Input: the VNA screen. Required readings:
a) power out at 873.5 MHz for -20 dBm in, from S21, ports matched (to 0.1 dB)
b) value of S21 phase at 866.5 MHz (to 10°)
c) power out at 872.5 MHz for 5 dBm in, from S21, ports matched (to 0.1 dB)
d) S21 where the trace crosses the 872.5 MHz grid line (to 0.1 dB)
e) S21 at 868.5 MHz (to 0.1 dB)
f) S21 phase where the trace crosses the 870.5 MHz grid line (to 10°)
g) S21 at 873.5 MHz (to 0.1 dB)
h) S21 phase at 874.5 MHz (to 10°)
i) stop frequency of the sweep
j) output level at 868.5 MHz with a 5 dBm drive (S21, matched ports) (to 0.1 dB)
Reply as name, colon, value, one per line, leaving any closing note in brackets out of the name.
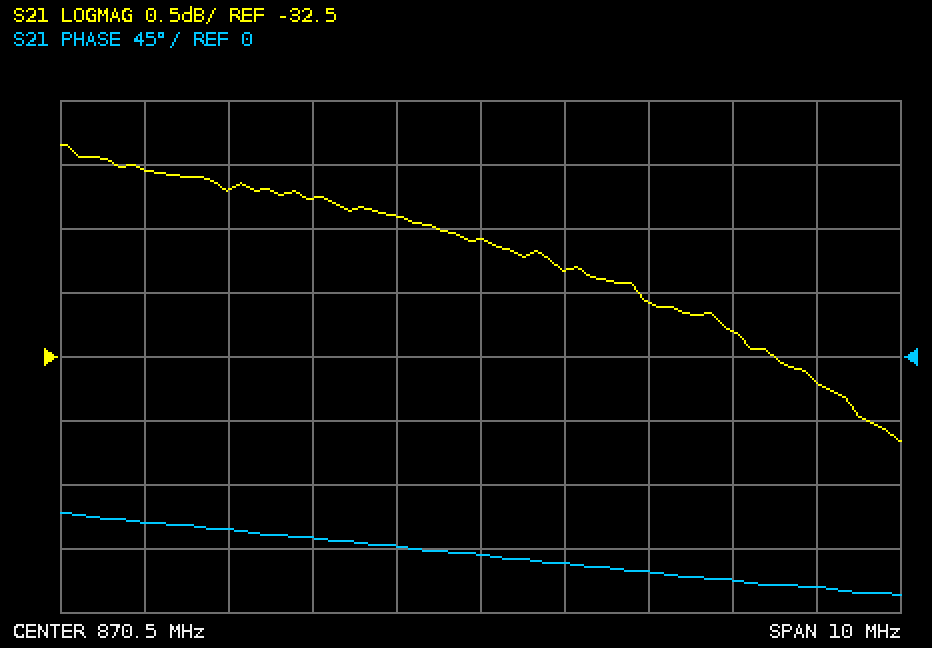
power out at 873.5 MHz for -20 dBm in, from S21, ports matched: -52.3 dBm
value of S21 phase at 866.5 MHz: -120°
power out at 872.5 MHz for 5 dBm in, from S21, ports matched: -27.1 dBm
S21 where the trace crosses the 872.5 MHz grid line: -32.1 dB
S21 at 868.5 MHz: -31.3 dB
S21 phase where the trace crosses the 870.5 MHz grid line: -140°
S21 at 873.5 MHz: -32.3 dB
S21 phase at 874.5 MHz: -160°
stop frequency of the sweep: 875.5 MHz
output level at 868.5 MHz with a 5 dBm drive (S21, matched ports): -26.3 dBm
